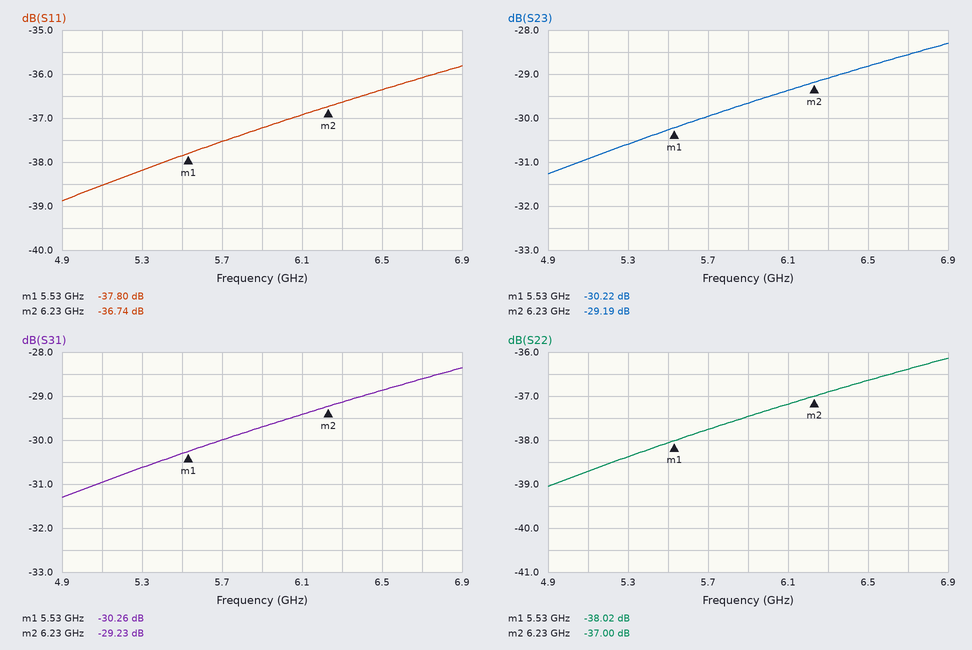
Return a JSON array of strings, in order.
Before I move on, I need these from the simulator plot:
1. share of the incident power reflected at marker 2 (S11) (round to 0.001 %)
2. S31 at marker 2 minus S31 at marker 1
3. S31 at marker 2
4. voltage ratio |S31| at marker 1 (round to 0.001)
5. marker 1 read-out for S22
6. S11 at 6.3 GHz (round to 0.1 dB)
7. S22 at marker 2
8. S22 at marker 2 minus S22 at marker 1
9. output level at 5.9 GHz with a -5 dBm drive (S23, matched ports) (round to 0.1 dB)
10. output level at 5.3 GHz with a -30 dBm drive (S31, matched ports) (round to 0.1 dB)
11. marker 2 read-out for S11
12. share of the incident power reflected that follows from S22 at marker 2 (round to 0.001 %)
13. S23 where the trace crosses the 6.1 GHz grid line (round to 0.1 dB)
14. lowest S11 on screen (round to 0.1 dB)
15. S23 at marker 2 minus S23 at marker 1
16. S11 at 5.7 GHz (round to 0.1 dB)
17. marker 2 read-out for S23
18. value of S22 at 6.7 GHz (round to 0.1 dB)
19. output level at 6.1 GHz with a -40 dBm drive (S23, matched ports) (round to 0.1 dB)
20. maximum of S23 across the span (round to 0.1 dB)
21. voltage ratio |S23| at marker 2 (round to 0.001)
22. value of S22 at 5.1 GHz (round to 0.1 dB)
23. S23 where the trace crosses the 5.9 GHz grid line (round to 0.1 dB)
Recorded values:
["0.021 %", "1.03 dB", "-29.23 dB", "0.031", "-38.02 dB", "-36.6 dB", "-37.00 dB", "1.02 dB", "-34.7 dBm", "-60.6 dBm", "-36.74 dB", "0.020 %", "-29.4 dB", "-38.9 dB", "1.03 dB", "-37.5 dB", "-29.19 dB", "-36.4 dB", "-69.4 dBm", "-28.3 dB", "0.035", "-38.7 dB", "-29.7 dB"]
